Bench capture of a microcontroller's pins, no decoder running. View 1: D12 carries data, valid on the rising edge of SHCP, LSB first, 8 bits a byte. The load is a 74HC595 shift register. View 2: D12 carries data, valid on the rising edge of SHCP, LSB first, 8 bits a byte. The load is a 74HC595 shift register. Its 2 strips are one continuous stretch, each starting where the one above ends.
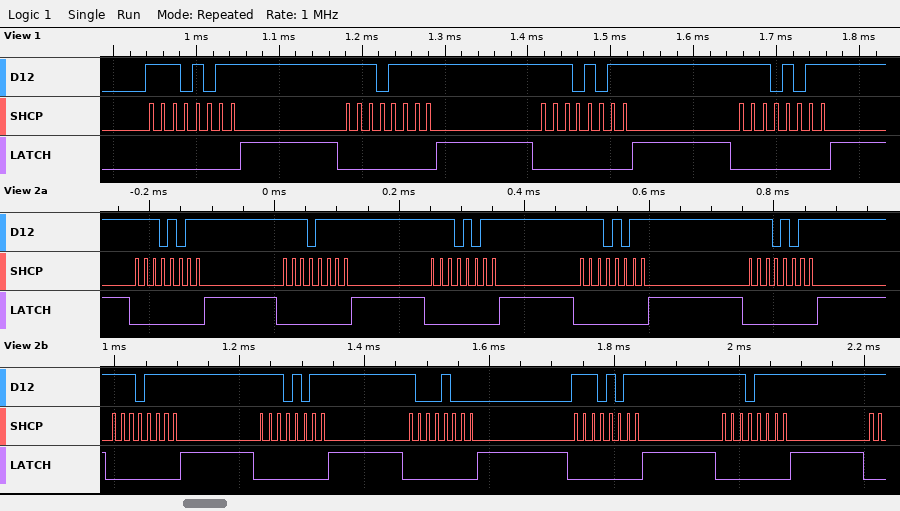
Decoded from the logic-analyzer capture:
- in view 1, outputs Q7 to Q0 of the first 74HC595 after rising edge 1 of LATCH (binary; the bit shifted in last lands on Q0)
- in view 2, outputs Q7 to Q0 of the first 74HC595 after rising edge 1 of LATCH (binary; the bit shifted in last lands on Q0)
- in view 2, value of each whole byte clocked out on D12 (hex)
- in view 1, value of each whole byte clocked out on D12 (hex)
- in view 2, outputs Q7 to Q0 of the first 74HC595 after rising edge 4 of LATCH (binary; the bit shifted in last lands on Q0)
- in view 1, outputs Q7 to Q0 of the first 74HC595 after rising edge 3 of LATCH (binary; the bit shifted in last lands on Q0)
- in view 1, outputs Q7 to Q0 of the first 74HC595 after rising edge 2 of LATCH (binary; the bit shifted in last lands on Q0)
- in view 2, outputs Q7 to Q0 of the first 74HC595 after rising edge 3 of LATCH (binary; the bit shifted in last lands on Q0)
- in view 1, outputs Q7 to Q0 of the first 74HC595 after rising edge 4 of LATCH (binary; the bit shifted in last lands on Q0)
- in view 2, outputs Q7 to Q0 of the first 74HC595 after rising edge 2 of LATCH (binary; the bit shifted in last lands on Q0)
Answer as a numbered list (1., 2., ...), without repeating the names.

1. 11101011
2. 11101011
3. D7 F7 D7 D7 D7 F7 D7 11 D7 F7
4. D7 F7 D7 D7
5. 11101011
6. 11101011
7. 11101111
8. 11101011
9. 11101011
10. 11101111
